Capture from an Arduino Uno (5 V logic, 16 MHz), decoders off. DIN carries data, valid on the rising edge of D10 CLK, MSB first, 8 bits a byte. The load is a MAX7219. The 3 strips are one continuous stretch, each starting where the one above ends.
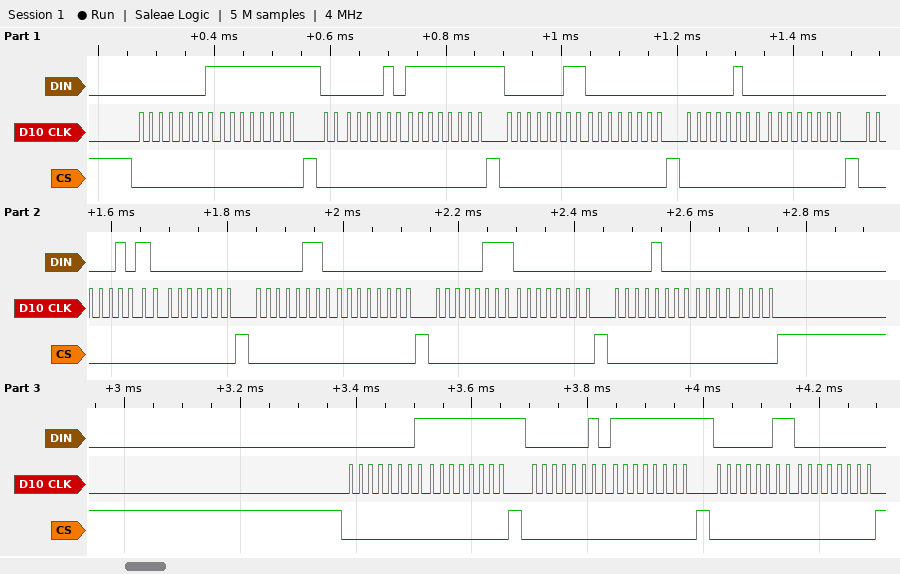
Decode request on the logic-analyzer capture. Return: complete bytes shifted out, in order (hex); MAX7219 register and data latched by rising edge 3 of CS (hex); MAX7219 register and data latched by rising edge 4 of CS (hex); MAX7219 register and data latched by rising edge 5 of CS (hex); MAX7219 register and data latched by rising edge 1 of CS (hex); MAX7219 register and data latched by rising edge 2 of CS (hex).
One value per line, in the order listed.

01 FF 02 FF 03 00 04 00 05 00 06 00 07 00 08 00 01 FF 02 FF 03 00
register 0x3, data 0x00
register 0x4, data 0x00
register 0x5, data 0x00
register 0x1, data 0xFF
register 0x2, data 0xFF
